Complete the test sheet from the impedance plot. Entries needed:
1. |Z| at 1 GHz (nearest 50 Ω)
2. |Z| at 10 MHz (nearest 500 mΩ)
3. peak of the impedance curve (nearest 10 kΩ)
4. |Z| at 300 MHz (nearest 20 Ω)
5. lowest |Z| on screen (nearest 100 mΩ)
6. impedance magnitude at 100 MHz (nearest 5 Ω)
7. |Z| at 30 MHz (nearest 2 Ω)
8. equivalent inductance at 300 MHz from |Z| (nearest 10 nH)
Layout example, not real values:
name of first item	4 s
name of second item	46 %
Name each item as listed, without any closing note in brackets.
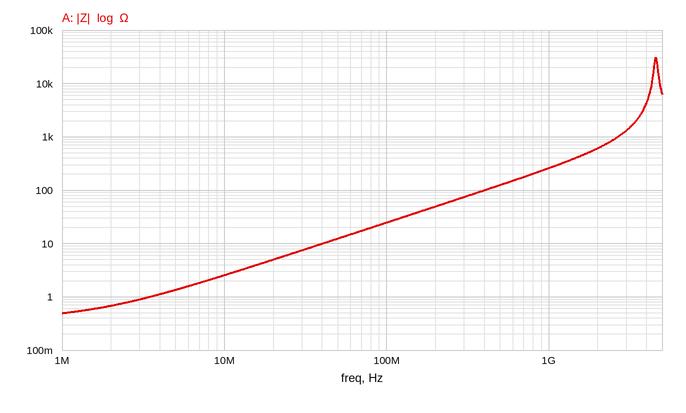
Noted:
|Z| at 1 GHz	250 Ω
|Z| at 10 MHz	2.5 Ω
peak of the impedance curve	30 kΩ
|Z| at 300 MHz	80 Ω
lowest |Z| on screen	500 mΩ
impedance magnitude at 100 MHz	25 Ω
|Z| at 30 MHz	8 Ω
equivalent inductance at 300 MHz from |Z|	40 nH
